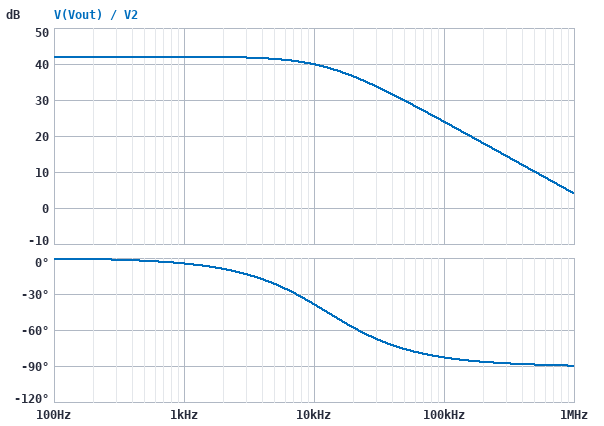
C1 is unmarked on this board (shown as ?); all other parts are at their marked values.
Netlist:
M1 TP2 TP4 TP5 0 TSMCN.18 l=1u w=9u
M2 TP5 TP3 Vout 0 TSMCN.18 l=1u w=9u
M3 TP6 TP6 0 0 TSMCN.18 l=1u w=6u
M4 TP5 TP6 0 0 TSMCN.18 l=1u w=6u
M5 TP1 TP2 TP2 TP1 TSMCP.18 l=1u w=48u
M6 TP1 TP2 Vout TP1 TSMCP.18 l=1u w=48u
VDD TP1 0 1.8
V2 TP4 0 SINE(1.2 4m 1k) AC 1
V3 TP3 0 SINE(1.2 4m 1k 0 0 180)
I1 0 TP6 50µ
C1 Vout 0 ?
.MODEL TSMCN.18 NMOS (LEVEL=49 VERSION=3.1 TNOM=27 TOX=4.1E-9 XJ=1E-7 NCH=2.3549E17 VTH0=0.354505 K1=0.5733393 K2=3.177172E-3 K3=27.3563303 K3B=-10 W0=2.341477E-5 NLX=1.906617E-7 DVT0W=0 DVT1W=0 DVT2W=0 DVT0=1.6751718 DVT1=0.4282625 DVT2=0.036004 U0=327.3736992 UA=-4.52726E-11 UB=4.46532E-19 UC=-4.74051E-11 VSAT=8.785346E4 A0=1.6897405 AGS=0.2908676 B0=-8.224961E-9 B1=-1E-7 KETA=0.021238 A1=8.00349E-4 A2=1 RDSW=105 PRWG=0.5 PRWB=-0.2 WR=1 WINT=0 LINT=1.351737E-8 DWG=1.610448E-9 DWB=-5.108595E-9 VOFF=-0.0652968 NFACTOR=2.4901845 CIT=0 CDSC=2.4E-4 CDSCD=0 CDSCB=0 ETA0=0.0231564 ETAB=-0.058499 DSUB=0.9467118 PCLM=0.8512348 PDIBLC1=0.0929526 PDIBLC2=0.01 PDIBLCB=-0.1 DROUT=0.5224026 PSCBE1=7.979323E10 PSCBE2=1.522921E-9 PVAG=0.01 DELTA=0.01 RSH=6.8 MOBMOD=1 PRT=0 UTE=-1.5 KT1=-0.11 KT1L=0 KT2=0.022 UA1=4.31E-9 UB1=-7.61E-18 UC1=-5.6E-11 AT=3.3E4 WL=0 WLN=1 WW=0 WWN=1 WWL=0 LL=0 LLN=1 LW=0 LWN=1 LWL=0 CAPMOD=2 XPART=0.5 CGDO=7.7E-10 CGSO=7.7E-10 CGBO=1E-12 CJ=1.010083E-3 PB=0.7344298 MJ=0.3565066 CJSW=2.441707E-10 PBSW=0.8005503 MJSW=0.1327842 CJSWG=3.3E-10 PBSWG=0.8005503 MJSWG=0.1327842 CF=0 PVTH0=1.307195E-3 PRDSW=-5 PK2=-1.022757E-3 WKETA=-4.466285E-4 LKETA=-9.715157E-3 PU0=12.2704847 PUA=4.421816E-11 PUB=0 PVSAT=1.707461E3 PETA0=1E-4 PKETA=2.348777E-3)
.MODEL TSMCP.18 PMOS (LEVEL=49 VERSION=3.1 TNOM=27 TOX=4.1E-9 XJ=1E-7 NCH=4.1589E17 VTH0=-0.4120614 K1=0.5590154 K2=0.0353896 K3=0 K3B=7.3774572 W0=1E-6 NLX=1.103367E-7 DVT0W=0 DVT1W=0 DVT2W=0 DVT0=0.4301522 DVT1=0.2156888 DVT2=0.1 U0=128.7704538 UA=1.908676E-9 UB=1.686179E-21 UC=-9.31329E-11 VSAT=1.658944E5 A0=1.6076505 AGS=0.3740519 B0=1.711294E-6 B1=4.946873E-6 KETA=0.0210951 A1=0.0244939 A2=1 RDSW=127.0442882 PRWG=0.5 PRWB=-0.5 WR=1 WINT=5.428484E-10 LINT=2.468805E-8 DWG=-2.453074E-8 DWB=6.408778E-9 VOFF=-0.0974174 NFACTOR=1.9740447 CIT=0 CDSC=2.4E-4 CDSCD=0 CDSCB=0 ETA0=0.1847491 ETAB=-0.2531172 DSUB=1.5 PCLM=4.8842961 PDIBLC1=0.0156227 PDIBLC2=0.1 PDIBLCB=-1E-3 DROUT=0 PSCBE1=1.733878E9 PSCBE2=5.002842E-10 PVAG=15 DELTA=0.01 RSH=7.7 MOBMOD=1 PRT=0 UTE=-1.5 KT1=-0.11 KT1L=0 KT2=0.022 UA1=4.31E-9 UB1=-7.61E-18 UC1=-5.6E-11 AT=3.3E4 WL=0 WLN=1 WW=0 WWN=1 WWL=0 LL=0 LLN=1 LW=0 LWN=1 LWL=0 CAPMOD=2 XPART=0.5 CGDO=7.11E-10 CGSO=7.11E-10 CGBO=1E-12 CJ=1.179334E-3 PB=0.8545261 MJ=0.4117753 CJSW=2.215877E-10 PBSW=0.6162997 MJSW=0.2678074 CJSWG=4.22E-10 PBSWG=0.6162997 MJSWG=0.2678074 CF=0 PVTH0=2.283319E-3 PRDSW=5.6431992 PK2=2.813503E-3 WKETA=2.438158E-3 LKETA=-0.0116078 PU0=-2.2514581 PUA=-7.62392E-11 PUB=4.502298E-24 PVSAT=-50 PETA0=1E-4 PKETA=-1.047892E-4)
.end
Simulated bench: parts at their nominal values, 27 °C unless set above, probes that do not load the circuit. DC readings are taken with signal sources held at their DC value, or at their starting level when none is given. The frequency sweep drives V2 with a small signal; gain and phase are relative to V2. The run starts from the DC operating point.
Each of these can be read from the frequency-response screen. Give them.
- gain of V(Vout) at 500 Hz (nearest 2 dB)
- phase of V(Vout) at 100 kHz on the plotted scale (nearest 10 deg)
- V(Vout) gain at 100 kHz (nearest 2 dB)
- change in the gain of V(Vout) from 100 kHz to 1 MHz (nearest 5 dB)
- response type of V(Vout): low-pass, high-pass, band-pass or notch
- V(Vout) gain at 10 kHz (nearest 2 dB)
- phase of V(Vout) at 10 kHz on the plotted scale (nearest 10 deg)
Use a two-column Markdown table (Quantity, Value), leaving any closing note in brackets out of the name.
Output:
| Quantity | Value |
|---|---|
| gain of V(Vout) at 500 Hz | 42 dB |
| phase of V(Vout) at 100 kHz on the plotted scale | -80 deg |
| V(Vout) gain at 100 kHz | 24 dB |
| change in the gain of V(Vout) from 100 kHz to 1 MHz | -20 dB |
| response type of V(Vout): low-pass, high-pass, band-pass or notch | low-pass |
| V(Vout) gain at 10 kHz | 40 dB |
| phase of V(Vout) at 10 kHz on the plotted scale | -40 deg |
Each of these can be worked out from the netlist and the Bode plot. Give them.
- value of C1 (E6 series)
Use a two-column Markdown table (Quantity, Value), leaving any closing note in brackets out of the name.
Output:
| Quantity | Value |
|---|---|
| value of C1 | 33 pF |
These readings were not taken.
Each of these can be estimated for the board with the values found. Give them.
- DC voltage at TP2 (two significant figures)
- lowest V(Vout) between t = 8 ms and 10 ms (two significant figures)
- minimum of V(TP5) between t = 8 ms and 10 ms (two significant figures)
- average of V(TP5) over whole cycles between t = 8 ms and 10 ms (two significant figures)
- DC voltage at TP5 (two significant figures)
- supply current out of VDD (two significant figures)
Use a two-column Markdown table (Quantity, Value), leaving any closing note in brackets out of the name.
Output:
| Quantity | Value |
|---|---|
| DC voltage at TP2 | 1.2 V |
| lowest V(Vout) between t = 8 ms and 10 ms | 650 mV |
| minimum of V(TP5) between t = 8 ms and 10 ms | 490 mV |
| average of V(TP5) over whole cycles between t = 8 ms and 10 ms | 490 mV |
| DC voltage at TP5 | 490 mV |
| supply current out of VDD | 49 µA |
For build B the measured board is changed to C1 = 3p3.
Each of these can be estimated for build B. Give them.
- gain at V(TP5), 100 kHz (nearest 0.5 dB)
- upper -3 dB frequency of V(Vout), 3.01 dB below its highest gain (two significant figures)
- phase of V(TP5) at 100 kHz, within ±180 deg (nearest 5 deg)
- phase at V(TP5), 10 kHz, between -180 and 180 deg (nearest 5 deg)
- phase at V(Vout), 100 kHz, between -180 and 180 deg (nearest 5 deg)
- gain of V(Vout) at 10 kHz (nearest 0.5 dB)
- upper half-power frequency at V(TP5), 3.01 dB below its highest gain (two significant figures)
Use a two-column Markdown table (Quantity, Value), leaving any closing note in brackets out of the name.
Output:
| Quantity | Value |
|---|---|
| gain at V(TP5), 100 kHz | -5.0 dB |
| upper -3 dB frequency of V(Vout), 3.01 dB below its highest gain | 120 kHz |
| phase of V(TP5) at 100 kHz, within ±180 deg | -15 deg |
| phase at V(TP5), 10 kHz, between -180 and 180 deg | 0 deg |
| phase at V(Vout), 100 kHz, between -180 and 180 deg | -40 deg |
| gain of V(Vout) at 10 kHz | 42.0 dB |
| upper half-power frequency at V(TP5), 3.01 dB below its highest gain | 230 kHz |
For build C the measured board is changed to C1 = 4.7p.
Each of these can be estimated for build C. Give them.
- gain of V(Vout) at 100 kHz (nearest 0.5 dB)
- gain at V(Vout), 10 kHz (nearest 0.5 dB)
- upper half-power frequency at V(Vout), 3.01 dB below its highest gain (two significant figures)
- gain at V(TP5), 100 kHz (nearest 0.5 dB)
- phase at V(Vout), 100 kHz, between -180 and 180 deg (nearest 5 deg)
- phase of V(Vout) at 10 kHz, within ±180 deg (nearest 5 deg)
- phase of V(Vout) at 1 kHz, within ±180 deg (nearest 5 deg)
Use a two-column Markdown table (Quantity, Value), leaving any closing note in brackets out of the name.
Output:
| Quantity | Value |
|---|---|
| gain of V(Vout) at 100 kHz | 38.5 dB |
| gain at V(Vout), 10 kHz | 42.0 dB |
| upper half-power frequency at V(Vout), 3.01 dB below its highest gain | 87 kHz |
| gain at V(TP5), 100 kHz | -5.5 dB |
| phase at V(Vout), 100 kHz, between -180 and 180 deg | -50 deg |
| phase of V(Vout) at 10 kHz, within ±180 deg | -5 deg |
| phase of V(Vout) at 1 kHz, within ±180 deg | 0 deg |
